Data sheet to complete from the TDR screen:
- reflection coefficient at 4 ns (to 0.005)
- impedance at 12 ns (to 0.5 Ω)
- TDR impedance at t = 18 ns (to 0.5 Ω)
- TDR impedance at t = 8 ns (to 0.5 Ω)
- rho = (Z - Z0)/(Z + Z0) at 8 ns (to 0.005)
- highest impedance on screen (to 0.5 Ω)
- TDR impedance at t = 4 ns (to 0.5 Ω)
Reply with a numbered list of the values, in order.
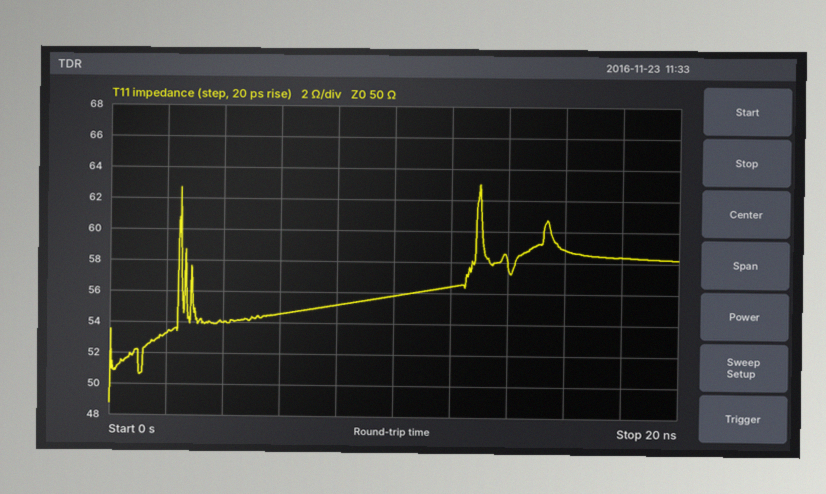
1. +0.040
2. 56.5 Ω
3. 58.5 Ω
4. 55.0 Ω
5. +0.050
6. 63.0 Ω
7. 54.0 Ω
